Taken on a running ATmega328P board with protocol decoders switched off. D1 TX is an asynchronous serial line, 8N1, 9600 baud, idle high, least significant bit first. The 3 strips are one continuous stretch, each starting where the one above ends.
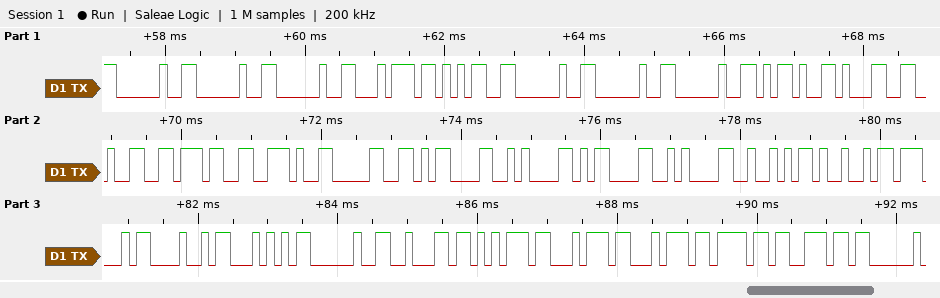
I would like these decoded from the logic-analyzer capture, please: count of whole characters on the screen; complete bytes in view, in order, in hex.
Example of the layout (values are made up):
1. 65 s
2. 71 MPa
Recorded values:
1. 30
2. 20 20 20 74 35 20 20 20 2D 31 32 37 2E 30 0D 0A 0D 0A 52 49 47 48 54 20 62 75 74 74 6F 6E
